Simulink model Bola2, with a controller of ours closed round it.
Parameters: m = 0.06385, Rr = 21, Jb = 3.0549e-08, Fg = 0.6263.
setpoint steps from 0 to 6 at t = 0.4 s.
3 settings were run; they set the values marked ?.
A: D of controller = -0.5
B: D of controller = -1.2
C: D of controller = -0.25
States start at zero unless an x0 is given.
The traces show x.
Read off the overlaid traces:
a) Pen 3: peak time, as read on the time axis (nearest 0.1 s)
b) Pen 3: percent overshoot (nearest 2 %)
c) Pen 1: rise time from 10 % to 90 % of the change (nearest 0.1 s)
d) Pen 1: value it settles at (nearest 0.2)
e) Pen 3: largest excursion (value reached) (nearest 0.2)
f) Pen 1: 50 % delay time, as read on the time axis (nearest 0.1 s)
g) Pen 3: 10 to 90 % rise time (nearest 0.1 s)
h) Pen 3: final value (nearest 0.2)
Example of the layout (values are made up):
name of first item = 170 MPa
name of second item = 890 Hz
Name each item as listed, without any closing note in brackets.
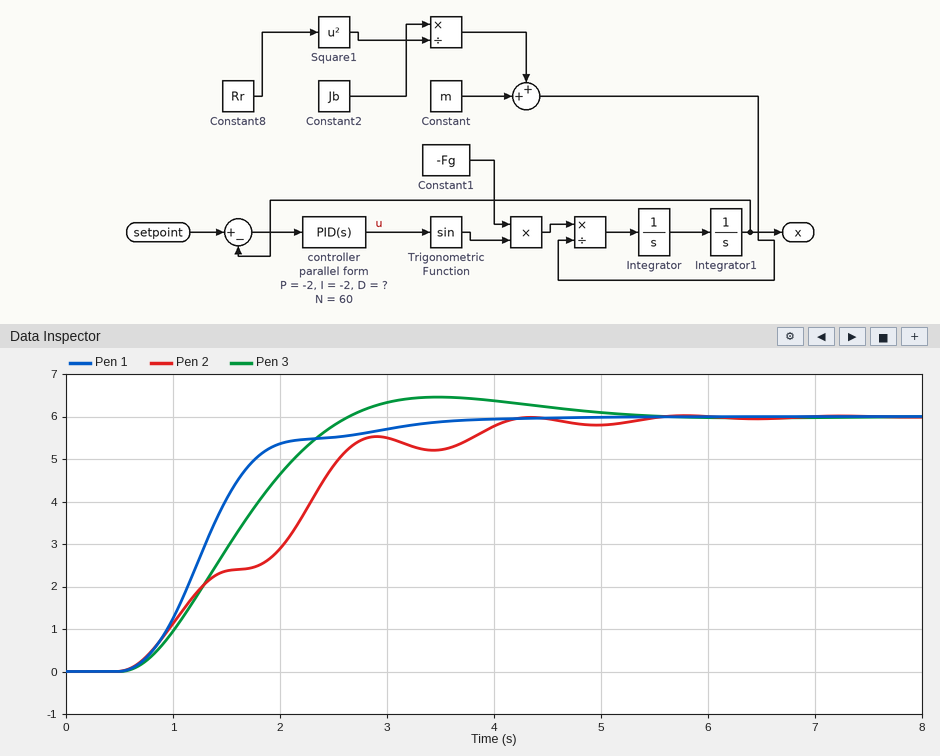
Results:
Pen 3: peak time, as read on the time axis = 3.5 s
Pen 3: percent overshoot = 8 %
Pen 1: rise time from 10 % to 90 % of the change = 1.2 s
Pen 1: value it settles at = 6.0
Pen 3: largest excursion (value reached) = 6.4
Pen 1: 50 % delay time, as read on the time axis = 1.3 s
Pen 3: 10 to 90 % rise time = 1.4 s
Pen 3: final value = 6.0
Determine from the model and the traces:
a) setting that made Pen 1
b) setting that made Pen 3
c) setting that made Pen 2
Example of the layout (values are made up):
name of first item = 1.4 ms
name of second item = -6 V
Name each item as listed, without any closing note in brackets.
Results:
setting that made Pen 1 = A
setting that made Pen 3 = B
setting that made Pen 2 = C
